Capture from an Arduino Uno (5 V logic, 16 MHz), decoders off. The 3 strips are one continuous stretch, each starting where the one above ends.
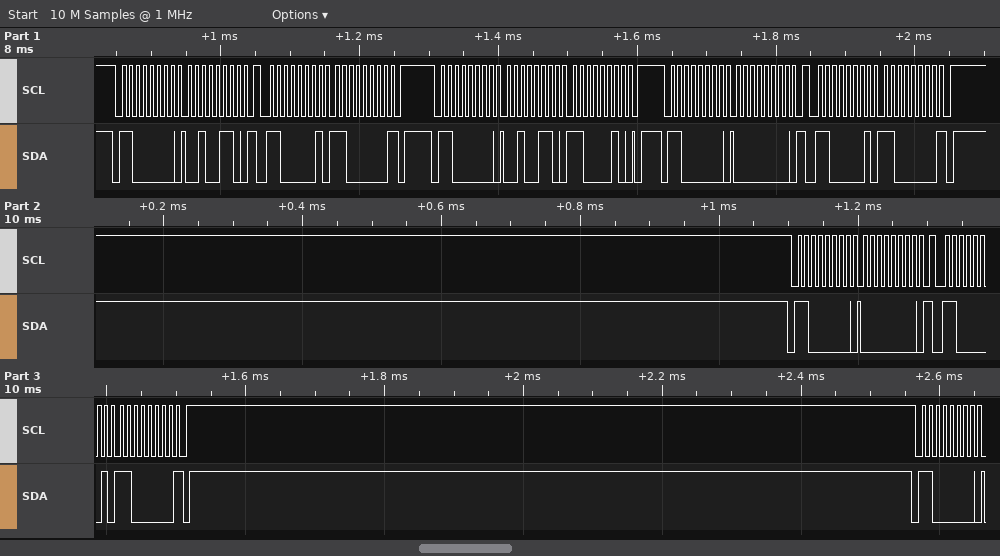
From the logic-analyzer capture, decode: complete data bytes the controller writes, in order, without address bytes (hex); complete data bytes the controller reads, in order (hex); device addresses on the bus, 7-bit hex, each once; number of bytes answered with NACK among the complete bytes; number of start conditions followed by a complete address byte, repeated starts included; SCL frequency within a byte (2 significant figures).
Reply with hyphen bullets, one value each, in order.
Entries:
- 26 26 C2 00 00
- C0 C0 C0
- 0x60
- 3
- 8
- 100 kHz
